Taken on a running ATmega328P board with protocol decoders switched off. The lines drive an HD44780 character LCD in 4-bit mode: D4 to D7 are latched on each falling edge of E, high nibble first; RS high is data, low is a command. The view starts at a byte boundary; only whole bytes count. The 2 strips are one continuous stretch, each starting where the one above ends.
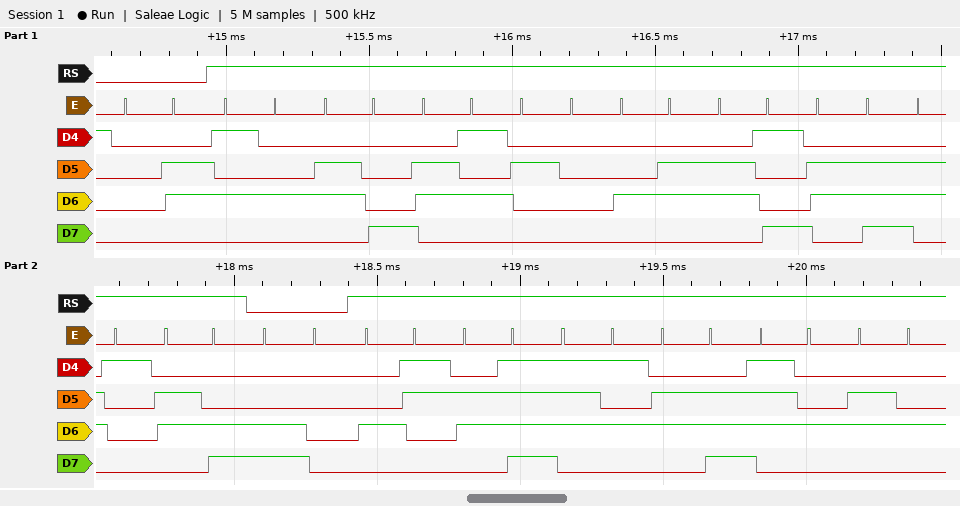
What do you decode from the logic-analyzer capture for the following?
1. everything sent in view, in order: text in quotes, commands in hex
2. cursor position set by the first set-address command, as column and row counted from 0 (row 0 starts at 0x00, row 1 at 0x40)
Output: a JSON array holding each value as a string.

["0x06 \"The Final\" 0xC0 \"Countd\"", "column 0, row 1"]
